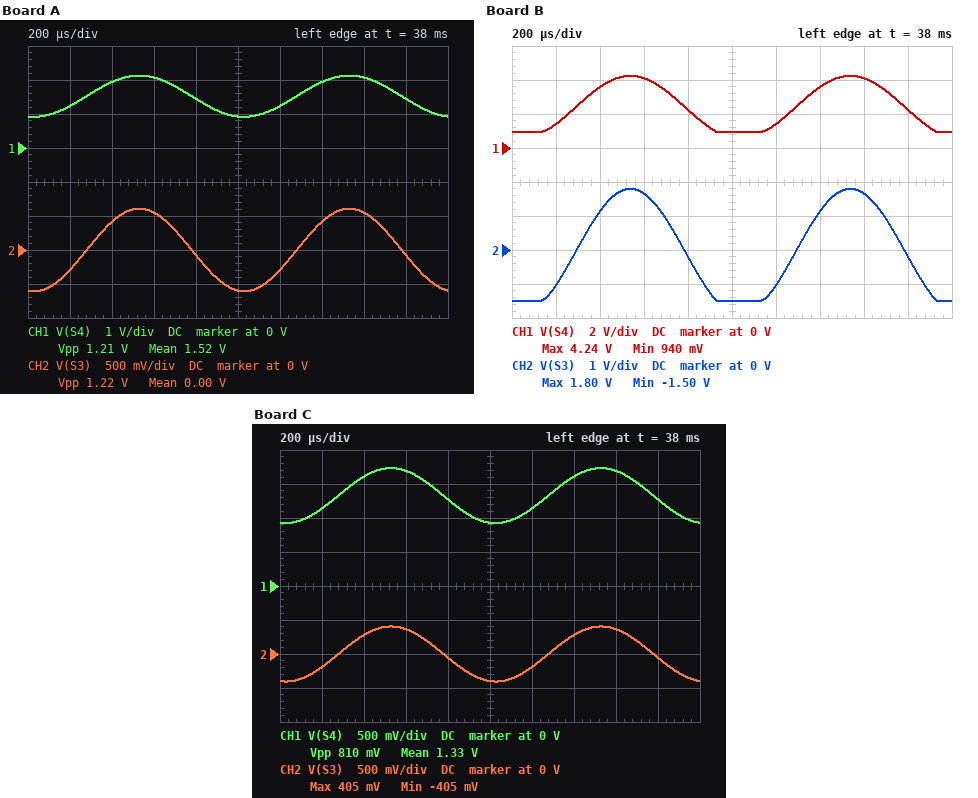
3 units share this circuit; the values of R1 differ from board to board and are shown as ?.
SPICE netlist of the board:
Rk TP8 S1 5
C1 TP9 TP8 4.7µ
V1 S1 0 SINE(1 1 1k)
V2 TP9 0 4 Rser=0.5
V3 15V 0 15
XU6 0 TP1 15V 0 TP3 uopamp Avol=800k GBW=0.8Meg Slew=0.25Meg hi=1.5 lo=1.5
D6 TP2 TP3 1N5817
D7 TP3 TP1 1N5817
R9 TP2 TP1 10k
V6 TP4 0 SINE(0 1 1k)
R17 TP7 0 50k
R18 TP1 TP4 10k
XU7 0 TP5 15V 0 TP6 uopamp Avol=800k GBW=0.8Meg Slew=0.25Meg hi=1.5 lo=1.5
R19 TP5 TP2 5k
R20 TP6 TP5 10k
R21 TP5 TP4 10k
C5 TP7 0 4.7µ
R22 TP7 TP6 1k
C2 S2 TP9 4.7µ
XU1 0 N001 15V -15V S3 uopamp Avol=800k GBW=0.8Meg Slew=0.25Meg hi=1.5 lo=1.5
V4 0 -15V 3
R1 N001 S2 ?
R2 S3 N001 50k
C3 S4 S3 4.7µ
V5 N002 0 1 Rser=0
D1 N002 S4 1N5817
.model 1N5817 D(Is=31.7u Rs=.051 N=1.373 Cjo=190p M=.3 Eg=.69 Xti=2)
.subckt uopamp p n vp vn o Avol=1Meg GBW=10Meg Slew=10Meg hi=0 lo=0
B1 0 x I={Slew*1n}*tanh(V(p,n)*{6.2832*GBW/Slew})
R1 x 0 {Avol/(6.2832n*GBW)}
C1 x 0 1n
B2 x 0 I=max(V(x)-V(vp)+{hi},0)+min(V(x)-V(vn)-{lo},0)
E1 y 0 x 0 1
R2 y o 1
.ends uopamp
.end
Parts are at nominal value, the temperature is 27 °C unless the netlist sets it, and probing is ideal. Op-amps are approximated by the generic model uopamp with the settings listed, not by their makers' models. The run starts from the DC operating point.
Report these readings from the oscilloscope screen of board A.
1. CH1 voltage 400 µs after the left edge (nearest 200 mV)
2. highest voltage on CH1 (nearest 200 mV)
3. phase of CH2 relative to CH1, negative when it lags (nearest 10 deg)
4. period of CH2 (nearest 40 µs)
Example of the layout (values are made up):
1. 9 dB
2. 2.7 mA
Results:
1. 2.0 V
2. 2.2 V
3. 0 deg
4. 1.00 ms
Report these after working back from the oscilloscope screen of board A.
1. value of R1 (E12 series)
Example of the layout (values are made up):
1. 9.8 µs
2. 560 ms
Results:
1. 1.2 kΩ
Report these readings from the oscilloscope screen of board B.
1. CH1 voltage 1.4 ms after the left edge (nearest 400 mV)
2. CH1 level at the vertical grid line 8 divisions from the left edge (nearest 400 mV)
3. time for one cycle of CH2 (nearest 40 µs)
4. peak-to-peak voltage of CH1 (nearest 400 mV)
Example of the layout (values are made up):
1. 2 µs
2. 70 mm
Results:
1. 3.6 V
2. 4.0 V
3. 1.00 ms
4. 3.2 V
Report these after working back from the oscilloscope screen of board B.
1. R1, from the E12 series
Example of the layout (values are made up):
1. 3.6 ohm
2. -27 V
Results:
1. 390 Ω
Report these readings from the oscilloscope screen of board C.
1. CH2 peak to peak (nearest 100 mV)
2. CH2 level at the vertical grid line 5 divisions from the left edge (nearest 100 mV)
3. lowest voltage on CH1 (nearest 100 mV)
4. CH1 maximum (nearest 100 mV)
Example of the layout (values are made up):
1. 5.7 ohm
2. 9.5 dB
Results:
1. 800 mV
2. -400 mV
3. 900 mV
4. 1.7 V
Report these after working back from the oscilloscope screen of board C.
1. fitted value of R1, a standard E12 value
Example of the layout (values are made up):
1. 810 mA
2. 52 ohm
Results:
1. 1.8 kΩ
